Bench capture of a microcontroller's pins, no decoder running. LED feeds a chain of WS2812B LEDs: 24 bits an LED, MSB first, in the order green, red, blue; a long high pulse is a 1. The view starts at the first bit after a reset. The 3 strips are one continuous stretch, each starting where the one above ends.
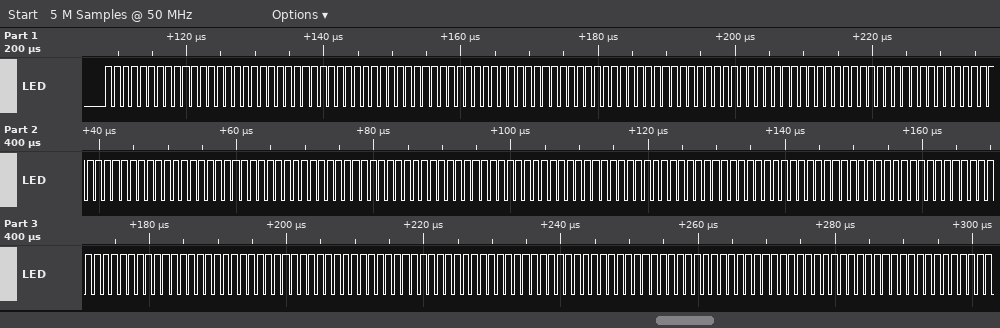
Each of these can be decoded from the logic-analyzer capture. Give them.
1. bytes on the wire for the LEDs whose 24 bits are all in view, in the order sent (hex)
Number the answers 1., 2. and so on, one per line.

1. FF FF FF FF FF FF FF FF FF FF FF FF FF FF FF FF FF FF FF FF FF FF FF FF FF FF FF FF FF FF FF FF FF FF FF FF FF FF FF
